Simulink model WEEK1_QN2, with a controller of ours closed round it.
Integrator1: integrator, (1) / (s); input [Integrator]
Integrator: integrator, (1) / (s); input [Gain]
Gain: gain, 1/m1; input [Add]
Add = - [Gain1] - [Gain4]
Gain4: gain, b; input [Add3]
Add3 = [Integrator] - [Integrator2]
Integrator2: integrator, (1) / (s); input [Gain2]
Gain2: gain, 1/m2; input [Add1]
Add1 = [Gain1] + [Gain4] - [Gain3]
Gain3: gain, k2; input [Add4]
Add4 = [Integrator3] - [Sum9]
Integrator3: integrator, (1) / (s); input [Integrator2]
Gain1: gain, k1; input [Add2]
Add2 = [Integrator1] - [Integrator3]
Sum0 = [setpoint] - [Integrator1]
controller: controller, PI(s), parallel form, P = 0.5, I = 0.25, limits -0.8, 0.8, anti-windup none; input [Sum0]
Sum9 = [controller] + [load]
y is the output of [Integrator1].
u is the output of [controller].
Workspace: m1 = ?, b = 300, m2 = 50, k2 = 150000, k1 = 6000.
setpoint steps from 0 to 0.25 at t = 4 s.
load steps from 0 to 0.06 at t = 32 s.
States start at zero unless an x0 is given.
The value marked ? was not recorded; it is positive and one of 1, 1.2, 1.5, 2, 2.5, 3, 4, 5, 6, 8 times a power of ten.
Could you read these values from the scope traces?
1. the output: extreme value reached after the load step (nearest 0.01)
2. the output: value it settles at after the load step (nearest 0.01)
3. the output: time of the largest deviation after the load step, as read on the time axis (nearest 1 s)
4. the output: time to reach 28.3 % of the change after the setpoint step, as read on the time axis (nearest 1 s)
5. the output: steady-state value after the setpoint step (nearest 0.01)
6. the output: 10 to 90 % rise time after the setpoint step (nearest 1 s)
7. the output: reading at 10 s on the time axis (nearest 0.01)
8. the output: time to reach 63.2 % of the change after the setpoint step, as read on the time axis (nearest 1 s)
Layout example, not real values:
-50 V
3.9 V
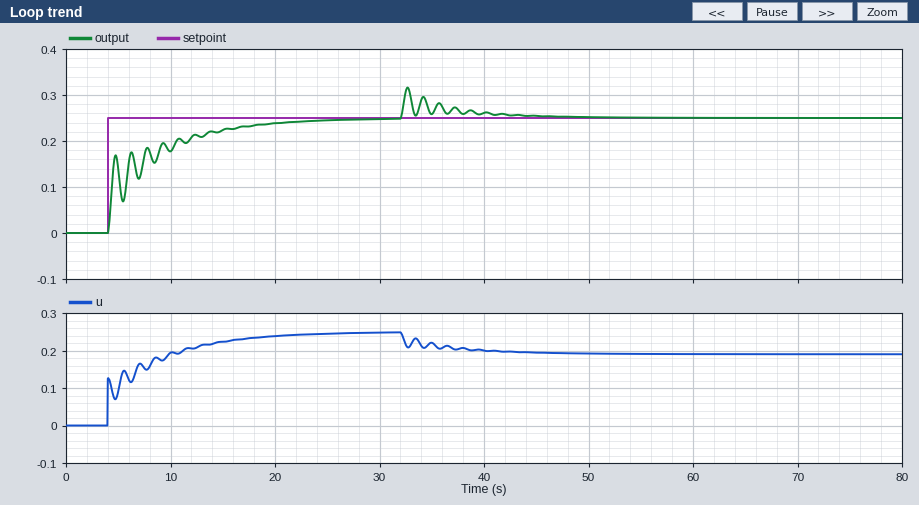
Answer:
0.32
0.25
33 s
4 s
0.25
11 s
0.18
5 s
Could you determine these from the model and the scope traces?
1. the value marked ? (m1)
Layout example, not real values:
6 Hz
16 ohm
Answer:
500
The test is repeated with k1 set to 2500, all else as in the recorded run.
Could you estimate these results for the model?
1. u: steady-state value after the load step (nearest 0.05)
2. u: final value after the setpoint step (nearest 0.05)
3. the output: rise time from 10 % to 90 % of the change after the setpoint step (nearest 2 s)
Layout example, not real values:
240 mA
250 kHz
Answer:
0.20
0.25
12 s
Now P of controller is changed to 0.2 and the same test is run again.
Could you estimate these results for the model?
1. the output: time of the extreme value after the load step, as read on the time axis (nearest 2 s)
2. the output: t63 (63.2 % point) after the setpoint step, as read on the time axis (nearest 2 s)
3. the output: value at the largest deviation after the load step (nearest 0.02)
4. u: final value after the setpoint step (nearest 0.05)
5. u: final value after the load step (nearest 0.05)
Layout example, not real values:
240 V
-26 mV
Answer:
32 s
8 s
0.34
0.25
0.20
